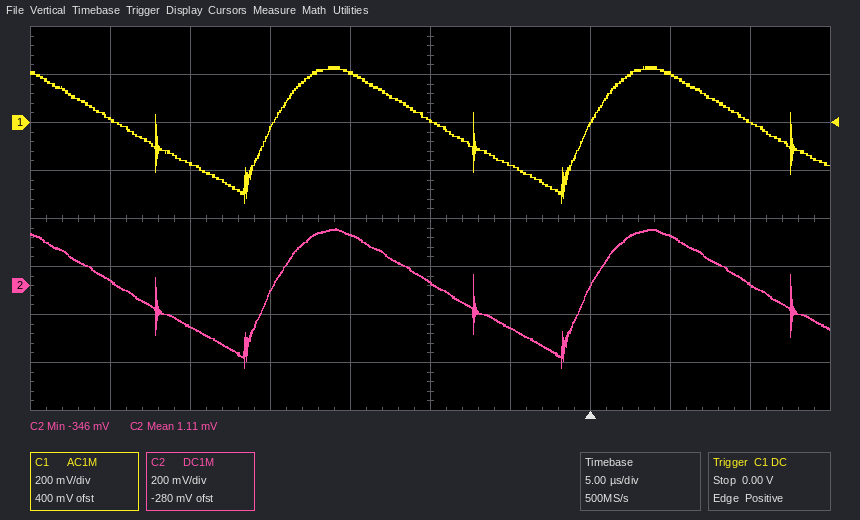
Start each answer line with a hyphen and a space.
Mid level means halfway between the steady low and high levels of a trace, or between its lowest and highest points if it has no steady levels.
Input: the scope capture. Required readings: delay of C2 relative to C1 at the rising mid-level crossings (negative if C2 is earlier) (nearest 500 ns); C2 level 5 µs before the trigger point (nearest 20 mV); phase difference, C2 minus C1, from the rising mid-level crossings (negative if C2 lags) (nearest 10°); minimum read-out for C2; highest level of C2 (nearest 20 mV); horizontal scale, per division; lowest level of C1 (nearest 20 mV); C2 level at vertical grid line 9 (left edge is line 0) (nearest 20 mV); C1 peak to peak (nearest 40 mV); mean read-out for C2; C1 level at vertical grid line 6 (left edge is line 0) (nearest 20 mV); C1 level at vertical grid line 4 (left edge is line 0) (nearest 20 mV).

- 0.0 µs
- -180 mV
- 0°
- -346 mV
- 240 mV
- 5 µs
- -340 mV
- 0 mV
- 560 mV
- 1.11 mV
- -180 mV
- 200 mV
